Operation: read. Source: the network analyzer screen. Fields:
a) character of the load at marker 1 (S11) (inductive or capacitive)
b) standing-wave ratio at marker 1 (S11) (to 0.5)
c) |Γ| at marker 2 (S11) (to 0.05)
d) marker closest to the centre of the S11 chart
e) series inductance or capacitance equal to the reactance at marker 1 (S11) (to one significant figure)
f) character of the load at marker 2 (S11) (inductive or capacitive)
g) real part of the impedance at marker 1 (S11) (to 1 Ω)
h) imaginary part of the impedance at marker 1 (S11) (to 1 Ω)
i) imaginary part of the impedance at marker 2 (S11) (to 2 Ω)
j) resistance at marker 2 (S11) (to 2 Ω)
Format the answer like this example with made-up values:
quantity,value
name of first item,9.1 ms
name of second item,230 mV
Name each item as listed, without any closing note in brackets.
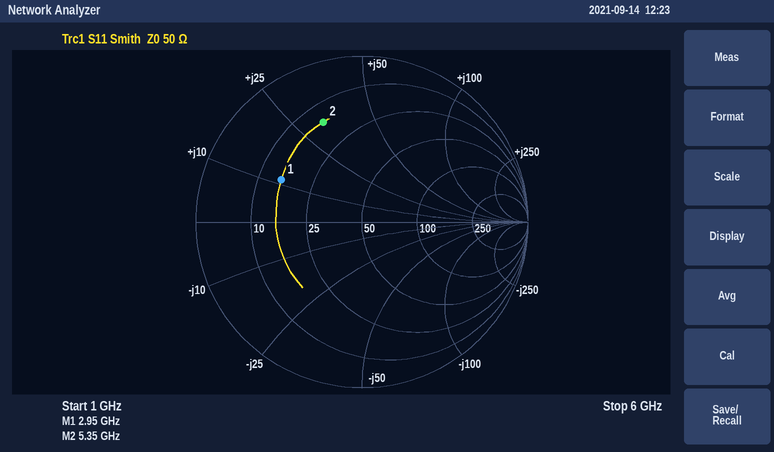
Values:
quantity,value
character of the load at marker 1 (S11),inductive
standing-wave ratio at marker 1 (S11),3.5
|Γ| at marker 2 (S11),0.65
marker closest to the centre of the S11 chart,marker 1
series inductance or capacitance equal to the reactance at marker 1 (S11),600 pH
character of the load at marker 2 (S11),inductive
real part of the impedance at marker 1 (S11),15 Ω
imaginary part of the impedance at marker 1 (S11),+11 Ω
imaginary part of the impedance at marker 2 (S11),+32 Ω
resistance at marker 2 (S11),16 Ω
